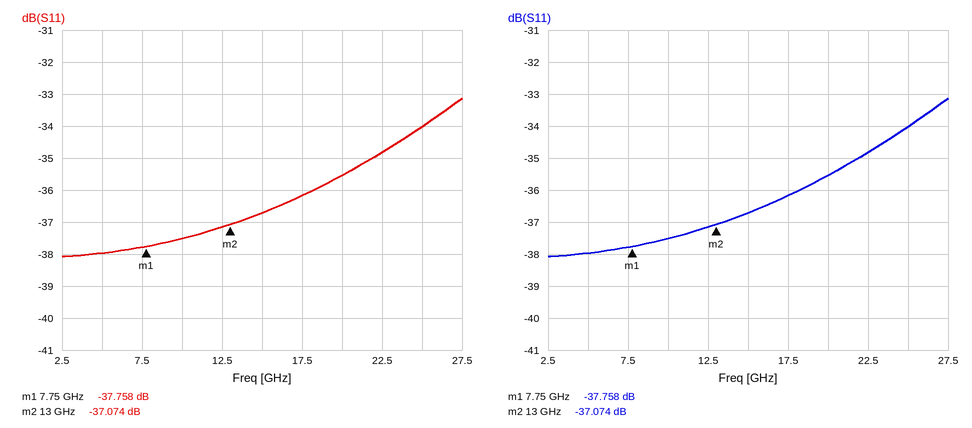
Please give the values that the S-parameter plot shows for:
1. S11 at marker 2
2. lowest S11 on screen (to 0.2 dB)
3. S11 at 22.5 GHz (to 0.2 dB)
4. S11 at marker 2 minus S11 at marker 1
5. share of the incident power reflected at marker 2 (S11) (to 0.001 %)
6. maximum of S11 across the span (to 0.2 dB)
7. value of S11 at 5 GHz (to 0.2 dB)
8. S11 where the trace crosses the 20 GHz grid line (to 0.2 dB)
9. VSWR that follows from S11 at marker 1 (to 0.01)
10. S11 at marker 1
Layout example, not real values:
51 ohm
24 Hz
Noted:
-37.074 dB
-38.0 dB
-34.8 dB
0.684 dB
0.020 %
-33.2 dB
-38.0 dB
-35.6 dB
1.03
-37.758 dB
